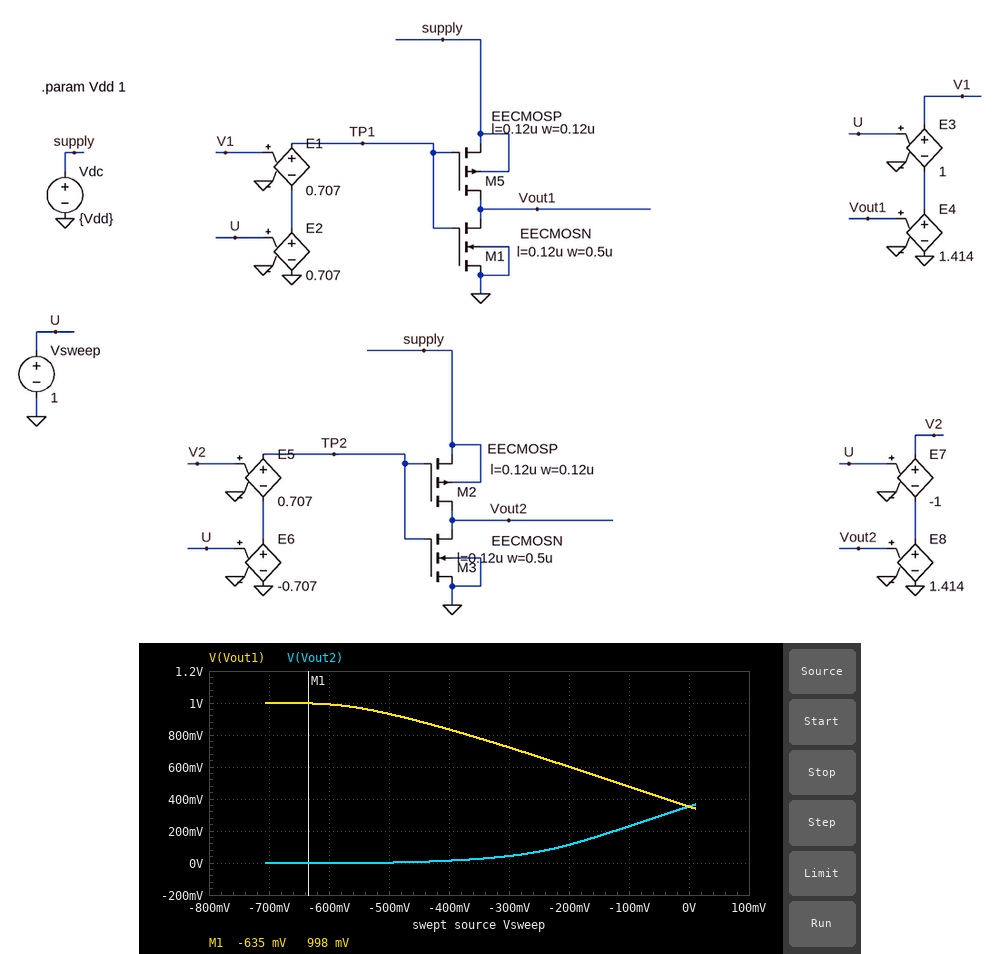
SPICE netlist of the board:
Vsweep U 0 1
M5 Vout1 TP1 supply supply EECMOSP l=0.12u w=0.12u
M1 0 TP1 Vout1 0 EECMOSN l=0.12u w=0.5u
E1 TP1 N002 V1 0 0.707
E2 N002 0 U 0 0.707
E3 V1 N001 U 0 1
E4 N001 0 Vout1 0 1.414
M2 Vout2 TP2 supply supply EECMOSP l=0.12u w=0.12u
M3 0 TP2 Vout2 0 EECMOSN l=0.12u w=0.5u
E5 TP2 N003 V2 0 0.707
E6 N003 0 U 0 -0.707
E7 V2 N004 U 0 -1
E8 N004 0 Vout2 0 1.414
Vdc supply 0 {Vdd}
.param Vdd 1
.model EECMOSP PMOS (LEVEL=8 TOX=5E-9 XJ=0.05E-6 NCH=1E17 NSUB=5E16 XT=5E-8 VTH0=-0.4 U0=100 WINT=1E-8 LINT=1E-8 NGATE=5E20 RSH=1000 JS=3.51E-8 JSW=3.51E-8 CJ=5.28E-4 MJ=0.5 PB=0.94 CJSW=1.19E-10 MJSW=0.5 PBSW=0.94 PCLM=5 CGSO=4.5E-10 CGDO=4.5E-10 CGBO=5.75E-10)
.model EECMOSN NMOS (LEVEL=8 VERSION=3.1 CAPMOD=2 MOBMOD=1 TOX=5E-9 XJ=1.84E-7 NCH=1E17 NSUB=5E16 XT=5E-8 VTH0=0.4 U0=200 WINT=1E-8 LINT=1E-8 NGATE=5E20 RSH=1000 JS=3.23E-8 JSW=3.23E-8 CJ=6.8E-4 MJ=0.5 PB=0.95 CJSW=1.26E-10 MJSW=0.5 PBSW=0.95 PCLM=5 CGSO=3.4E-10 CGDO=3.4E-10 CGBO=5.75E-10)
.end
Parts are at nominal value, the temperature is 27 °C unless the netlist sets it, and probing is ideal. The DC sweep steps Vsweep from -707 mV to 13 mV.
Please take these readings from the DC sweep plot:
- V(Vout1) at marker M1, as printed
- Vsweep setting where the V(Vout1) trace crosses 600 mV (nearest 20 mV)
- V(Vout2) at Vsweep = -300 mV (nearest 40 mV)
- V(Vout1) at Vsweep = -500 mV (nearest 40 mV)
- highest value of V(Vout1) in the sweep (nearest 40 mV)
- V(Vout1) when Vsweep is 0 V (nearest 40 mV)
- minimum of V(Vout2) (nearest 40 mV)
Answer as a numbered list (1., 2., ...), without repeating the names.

1. 998 mV
2. -200 mV
3. 40 mV
4. 920 mV
5. 1.00 V
6. 360 mV
7. 0 V
